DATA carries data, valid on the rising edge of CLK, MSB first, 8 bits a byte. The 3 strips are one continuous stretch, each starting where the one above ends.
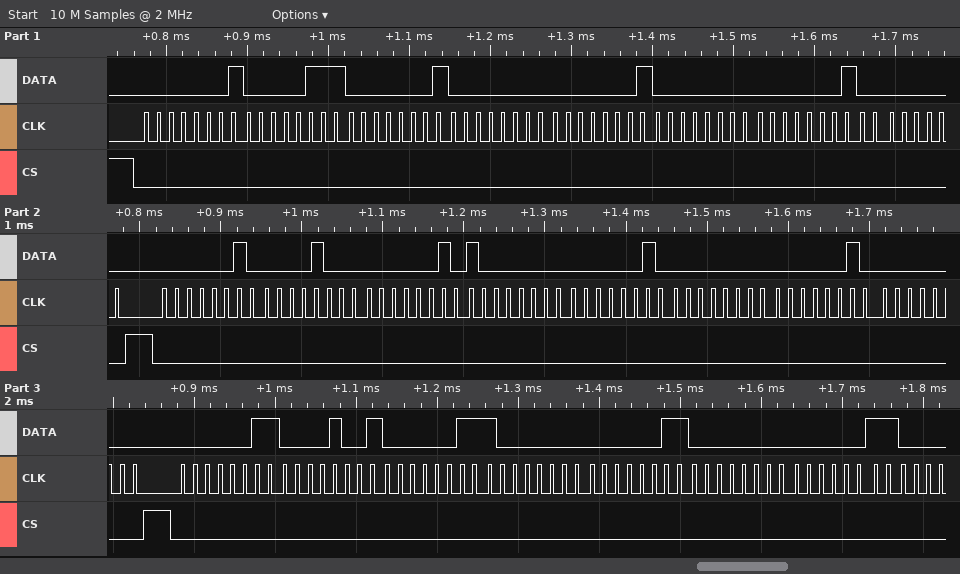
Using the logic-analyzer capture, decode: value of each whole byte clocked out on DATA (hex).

0x01 0x07 0x01 0x00 0x01 0x00 0x01 0x00 0x02 0x08 0x02 0x80 0x02 0x00 0x02 0x00 0x03 0x09 0x03 0x80 0x03 0x00 0x03
